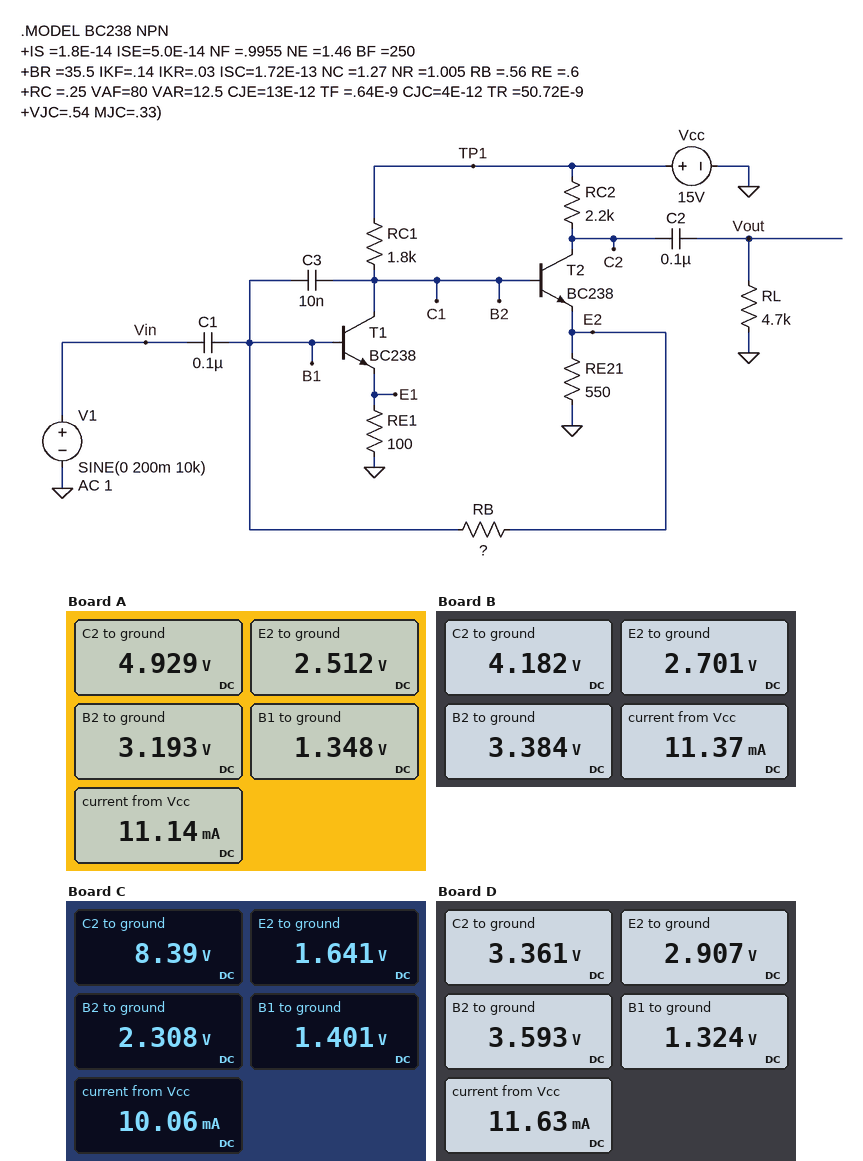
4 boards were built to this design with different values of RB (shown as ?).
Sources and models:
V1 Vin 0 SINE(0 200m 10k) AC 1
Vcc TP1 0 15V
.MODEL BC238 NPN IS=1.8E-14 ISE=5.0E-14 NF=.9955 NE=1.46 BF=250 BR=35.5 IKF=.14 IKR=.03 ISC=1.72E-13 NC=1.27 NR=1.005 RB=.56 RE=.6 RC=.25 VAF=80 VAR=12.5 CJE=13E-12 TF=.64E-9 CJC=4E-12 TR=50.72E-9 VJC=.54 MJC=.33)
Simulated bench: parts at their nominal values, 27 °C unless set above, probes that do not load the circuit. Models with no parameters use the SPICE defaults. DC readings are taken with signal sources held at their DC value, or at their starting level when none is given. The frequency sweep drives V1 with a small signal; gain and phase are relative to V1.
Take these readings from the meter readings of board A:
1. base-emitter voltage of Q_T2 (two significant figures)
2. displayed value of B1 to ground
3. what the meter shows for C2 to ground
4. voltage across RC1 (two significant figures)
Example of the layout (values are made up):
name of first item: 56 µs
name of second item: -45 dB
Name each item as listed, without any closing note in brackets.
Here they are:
base-emitter voltage of Q_T2: 680 mV
displayed value of B1 to ground: 1.348 V
what the meter shows for C2 to ground: 4.929 V
voltage across RC1: 12 V
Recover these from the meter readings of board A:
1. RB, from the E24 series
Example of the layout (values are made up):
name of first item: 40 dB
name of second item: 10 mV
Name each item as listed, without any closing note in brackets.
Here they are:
RB, from the E24 series: 36 kΩ
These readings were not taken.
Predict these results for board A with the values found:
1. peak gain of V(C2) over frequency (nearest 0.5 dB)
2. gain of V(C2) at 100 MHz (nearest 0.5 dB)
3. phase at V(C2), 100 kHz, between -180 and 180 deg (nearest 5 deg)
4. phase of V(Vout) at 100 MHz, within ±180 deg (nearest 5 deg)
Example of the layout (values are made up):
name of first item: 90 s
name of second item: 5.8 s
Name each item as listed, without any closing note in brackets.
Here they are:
peak gain of V(C2) over frequency: 24.5 dB
gain of V(C2) at 100 MHz: 4.0 dB
phase at V(C2), 100 kHz, between -180 and 180 deg: -110 deg
phase of V(Vout) at 100 MHz, within ±180 deg: 55 deg
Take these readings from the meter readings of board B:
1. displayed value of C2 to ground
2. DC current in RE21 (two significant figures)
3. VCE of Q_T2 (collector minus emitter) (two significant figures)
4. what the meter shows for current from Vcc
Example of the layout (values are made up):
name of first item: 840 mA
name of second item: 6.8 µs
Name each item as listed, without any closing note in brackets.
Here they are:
displayed value of C2 to ground: 4.182 V
DC current in RE21: 4.9 mA
VCE of Q_T2 (collector minus emitter): 1.5 V
what the meter shows for current from Vcc: 11.37 mA
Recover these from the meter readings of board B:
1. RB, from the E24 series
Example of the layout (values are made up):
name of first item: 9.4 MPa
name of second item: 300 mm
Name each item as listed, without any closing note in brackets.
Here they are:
RB, from the E24 series: 43 kΩ
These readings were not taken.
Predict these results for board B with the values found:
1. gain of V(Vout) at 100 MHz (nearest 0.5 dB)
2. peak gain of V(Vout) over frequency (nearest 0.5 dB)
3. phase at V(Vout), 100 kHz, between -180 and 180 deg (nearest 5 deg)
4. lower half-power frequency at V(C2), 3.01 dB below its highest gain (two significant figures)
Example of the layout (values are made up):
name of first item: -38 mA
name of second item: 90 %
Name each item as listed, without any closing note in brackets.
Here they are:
gain of V(Vout) at 100 MHz: 3.5 dB
peak gain of V(Vout) over frequency: 24.0 dB
phase at V(Vout), 100 kHz, between -180 and 180 deg: -110 deg
lower half-power frequency at V(C2), 3.01 dB below its highest gain: 170 Hz
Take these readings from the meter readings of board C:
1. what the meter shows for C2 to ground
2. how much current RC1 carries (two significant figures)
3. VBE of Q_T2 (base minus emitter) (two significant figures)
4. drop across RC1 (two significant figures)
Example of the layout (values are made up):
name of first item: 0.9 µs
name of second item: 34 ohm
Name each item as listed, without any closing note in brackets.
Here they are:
what the meter shows for C2 to ground: 8.39 V
how much current RC1 carries: 7.1 mA
VBE of Q_T2 (base minus emitter): 670 mV
drop across RC1: 13 V
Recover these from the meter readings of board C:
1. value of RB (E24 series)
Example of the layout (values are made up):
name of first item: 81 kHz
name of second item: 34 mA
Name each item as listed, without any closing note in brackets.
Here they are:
value of RB: 6.8 kΩ
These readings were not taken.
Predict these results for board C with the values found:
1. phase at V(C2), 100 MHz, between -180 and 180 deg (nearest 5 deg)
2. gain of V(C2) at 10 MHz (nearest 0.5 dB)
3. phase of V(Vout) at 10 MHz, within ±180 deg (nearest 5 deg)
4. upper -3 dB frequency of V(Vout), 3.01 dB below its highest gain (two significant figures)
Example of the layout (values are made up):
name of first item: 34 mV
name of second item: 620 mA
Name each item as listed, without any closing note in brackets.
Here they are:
phase at V(C2), 100 MHz, between -180 and 180 deg: 70 deg
gain of V(C2) at 10 MHz: 8.5 dB
phase of V(Vout) at 10 MHz, within ±180 deg: 165 deg
upper -3 dB frequency of V(Vout), 3.01 dB below its highest gain: 27 kHz
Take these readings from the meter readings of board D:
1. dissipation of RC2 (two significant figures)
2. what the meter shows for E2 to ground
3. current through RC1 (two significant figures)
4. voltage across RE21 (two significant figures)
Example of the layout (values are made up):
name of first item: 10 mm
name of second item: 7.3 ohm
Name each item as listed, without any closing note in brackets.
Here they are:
dissipation of RC2: 62 mW
what the meter shows for E2 to ground: 2.907 V
current through RC1: 6.3 mA
voltage across RE21: 2.9 V
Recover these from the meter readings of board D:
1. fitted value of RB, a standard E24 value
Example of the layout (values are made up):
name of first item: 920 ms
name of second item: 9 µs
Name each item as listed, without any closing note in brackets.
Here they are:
fitted value of RB, a standard E24 value: 51 kΩ
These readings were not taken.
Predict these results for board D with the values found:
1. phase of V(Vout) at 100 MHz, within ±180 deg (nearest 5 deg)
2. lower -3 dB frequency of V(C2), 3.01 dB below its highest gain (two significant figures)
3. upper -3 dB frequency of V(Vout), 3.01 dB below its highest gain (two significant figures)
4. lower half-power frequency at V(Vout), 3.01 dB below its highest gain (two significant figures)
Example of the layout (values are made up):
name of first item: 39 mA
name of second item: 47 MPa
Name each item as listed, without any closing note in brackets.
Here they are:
phase of V(Vout) at 100 MHz, within ±180 deg: 35 deg
lower -3 dB frequency of V(C2), 3.01 dB below its highest gain: 140 Hz
upper -3 dB frequency of V(Vout), 3.01 dB below its highest gain: 26 kHz
lower half-power frequency at V(Vout), 3.01 dB below its highest gain: 350 Hz
